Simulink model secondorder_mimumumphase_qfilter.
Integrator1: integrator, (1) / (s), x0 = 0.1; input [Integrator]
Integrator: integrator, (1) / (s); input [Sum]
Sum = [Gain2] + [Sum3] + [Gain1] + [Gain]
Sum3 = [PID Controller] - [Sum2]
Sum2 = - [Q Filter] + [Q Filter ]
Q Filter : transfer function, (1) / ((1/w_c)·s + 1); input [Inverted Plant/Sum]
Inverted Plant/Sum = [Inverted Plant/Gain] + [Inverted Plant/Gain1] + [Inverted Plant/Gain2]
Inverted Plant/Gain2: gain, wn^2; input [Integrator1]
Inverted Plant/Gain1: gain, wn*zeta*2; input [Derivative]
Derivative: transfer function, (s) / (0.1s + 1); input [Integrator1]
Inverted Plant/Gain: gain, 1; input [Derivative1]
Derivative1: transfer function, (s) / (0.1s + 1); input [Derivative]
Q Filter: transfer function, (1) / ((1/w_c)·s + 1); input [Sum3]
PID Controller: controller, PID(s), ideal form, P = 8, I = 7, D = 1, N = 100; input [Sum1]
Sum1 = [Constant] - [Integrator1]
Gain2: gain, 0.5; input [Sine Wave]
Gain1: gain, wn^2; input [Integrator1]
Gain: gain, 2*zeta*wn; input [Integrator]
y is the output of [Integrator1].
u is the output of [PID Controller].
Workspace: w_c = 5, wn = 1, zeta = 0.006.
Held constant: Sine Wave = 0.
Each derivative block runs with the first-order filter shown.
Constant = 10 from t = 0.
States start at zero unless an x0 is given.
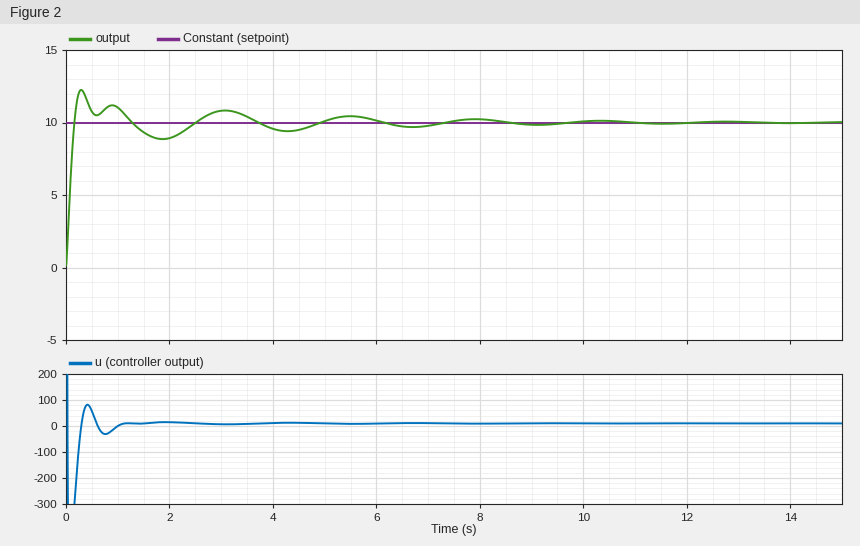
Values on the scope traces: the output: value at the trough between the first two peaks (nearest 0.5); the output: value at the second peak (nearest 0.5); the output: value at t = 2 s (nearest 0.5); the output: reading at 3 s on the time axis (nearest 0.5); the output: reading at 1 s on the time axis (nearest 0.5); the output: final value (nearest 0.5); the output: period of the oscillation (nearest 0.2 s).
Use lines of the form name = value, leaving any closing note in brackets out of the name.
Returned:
the output: value at the trough between the first two peaks = 9.0
the output: value at the second peak = 11.0
the output: value at t = 2 s = 9.0
the output: reading at 3 s on the time axis = 11.0
the output: reading at 1 s on the time axis = 11.0
the output: final value = 10.0
the output: period of the oscillation = 2.8 s
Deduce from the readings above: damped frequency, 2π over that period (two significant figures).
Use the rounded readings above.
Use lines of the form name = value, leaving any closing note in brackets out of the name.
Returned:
damped frequency, 2π over that period = 2.2 rad/s
